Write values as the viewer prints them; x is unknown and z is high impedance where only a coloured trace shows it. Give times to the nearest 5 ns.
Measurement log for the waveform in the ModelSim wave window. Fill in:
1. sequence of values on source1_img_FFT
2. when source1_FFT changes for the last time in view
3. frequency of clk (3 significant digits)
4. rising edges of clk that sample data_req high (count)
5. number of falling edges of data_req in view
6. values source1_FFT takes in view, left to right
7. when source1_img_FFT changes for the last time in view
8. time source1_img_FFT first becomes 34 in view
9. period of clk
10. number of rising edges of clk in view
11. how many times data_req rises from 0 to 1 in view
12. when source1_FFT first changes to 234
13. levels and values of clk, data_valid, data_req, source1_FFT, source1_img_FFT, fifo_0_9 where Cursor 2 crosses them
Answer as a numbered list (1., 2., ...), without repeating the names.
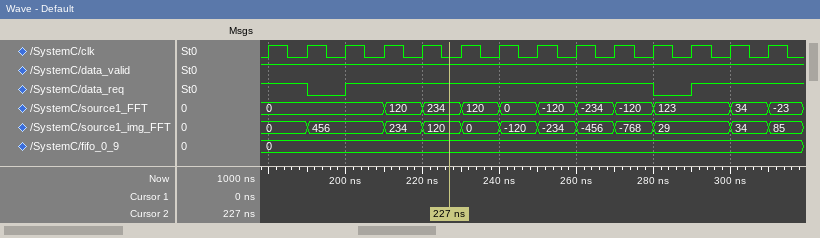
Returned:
1. 0, 456, 234, 120, 0, -120, -234, -456, -768, 29, 34, 85
2. 310 ns
3. 100 MHz
4. 12
5. 2
6. 0, 120, 234, 120, 0, -120, -234, -120, 123, 34, -23
7. 310 ns
8. 300 ns
9. 10 ns
10. 14
11. 2
12. 220 ns
13. clk=0, data_valid=1, data_req=1, source1_FFT=234, source1_img_FFT=120, fifo_0_9=0
